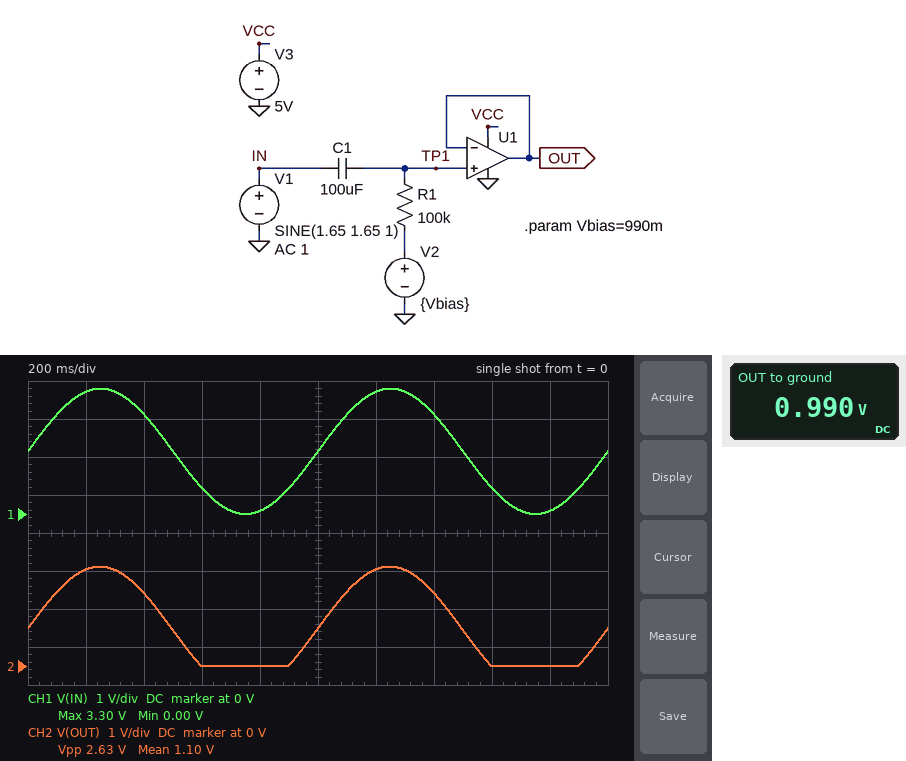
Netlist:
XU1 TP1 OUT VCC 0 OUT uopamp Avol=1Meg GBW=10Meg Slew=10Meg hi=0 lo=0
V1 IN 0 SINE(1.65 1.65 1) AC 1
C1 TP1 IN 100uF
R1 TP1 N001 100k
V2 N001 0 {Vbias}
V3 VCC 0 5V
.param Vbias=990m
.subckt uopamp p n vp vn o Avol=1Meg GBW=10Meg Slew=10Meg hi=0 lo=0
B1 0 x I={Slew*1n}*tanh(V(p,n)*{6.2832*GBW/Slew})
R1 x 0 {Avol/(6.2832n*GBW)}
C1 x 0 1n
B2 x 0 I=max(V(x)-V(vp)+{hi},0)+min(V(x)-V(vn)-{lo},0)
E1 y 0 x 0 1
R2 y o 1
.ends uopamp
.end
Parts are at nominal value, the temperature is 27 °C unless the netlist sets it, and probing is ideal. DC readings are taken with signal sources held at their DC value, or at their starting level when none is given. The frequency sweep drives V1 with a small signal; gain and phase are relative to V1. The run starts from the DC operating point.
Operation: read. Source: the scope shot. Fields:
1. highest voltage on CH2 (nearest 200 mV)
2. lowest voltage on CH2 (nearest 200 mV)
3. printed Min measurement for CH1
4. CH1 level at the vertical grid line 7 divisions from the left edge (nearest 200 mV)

2.6 V
0 V
0.00 V
2.6 V
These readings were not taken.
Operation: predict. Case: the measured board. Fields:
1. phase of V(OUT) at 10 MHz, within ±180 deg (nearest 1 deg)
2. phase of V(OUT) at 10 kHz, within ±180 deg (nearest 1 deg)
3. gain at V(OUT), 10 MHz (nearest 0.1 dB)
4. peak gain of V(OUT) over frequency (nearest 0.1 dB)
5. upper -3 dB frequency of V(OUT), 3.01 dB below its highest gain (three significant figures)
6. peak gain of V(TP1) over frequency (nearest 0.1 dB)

-45 deg
0 deg
-3.0 dB
0 dB
10.0 MHz
0 dB
